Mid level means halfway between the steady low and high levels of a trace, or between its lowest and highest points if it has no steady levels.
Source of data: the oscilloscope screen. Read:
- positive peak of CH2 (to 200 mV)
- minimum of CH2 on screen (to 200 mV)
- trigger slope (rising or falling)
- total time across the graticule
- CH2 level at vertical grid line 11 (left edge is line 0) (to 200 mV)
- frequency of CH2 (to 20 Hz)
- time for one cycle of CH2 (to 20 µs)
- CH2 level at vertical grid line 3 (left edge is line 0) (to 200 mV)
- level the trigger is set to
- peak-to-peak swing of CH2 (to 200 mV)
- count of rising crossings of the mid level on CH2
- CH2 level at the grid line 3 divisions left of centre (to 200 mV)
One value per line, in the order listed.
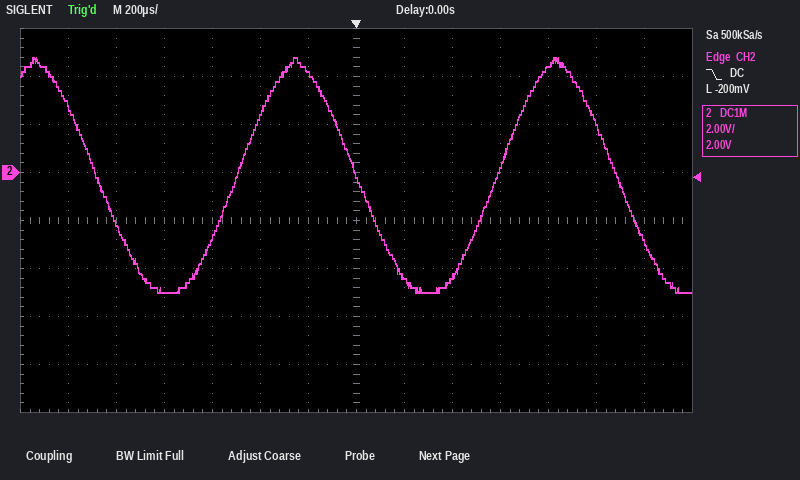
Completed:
4.8 V
-5.0 V
falling
2.8 ms
4.4 V
920 Hz
1.08 ms
-5.0 V
-200 mV
9.8 V
2
-2.8 V
